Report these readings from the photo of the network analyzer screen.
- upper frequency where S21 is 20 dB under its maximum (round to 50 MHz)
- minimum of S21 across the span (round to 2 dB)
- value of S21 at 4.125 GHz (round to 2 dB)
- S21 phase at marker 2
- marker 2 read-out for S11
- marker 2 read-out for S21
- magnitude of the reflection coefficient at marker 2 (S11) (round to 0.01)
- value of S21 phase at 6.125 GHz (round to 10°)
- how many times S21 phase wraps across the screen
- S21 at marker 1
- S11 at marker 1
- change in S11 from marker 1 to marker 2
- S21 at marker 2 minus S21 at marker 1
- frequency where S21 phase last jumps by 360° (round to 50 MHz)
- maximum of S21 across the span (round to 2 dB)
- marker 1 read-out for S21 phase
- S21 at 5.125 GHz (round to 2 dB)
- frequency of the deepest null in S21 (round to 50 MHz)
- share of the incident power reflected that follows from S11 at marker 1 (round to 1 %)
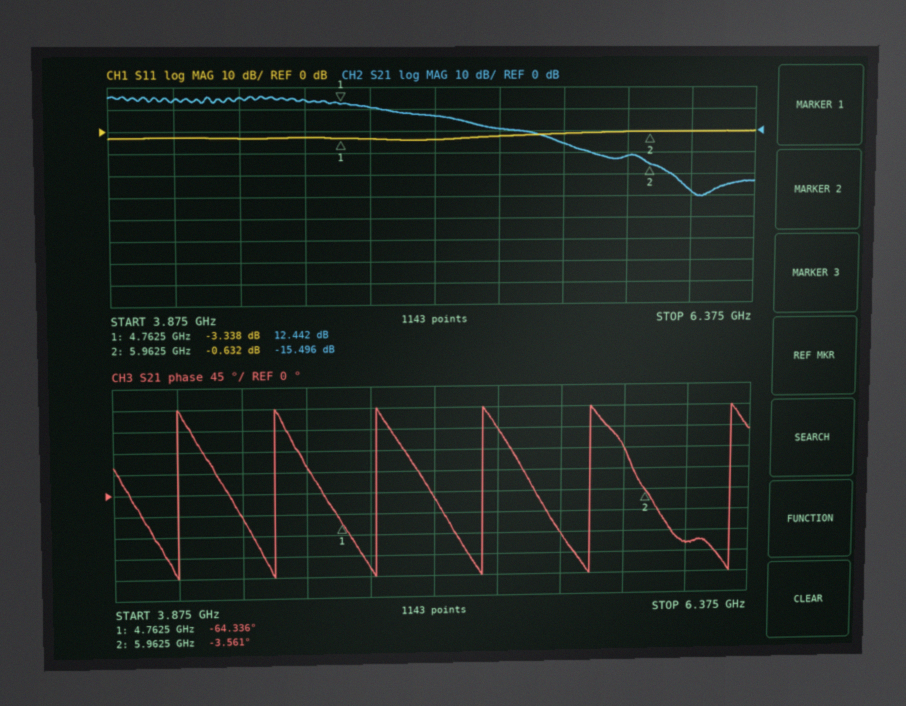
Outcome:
5.60 GHz
-30 dB
14 dB
-3.561°
-0.632 dB
-15.496 dB
0.93
-120°
6
12.442 dB
-3.338 dB
2.706 dB
-27.938 dB
6.30 GHz
16 dB
-64.336°
6 dB
6.15 GHz
46 %
